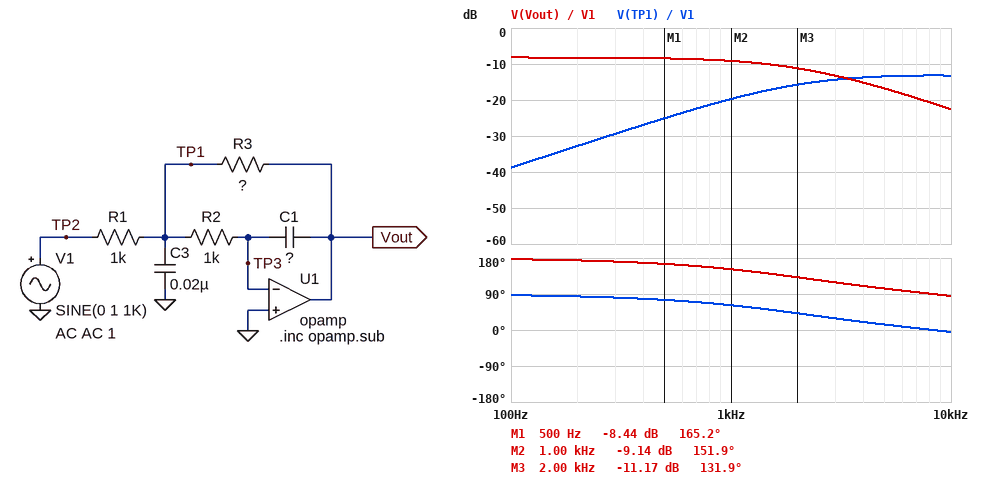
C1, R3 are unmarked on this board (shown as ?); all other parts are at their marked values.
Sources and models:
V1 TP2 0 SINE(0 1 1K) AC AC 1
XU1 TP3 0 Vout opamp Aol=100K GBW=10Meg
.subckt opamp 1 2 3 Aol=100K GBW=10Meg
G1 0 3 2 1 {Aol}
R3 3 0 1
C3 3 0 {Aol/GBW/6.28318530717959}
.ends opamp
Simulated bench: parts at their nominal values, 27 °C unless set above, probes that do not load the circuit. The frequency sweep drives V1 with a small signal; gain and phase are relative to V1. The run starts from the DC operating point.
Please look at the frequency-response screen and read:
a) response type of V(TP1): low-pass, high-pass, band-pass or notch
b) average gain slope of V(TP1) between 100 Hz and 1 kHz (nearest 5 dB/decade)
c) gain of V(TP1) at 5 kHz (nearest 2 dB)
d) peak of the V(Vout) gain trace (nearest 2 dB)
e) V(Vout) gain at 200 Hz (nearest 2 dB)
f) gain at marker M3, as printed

high-pass
20 dB/decade
-14 dB
-8 dB
-8 dB
-11.17 dB
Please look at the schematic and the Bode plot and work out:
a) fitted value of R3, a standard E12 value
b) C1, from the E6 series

390 Ω
47 nF
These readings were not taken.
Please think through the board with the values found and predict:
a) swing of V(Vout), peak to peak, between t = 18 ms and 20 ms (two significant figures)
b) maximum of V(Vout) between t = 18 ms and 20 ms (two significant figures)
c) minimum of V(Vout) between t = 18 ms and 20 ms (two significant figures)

700 mV
350 mV
-350 mV
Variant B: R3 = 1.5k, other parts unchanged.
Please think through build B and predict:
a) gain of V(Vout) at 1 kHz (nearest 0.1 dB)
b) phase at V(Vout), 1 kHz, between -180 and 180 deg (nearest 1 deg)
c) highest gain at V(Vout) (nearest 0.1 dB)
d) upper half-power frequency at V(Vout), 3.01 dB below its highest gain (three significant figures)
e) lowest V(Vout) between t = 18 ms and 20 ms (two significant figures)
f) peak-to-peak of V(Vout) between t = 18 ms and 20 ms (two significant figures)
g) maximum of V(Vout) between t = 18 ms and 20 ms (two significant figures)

-0.1 dB
129 deg
3.5 dB
882 Hz
-990 mV
2.0 V
990 mV
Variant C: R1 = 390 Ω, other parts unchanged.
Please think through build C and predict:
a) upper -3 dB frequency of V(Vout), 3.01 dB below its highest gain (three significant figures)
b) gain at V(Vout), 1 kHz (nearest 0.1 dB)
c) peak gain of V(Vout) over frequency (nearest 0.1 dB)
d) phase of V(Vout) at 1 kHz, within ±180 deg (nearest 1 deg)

1.46 kHz
-1.7 dB
0 dB
144 deg
